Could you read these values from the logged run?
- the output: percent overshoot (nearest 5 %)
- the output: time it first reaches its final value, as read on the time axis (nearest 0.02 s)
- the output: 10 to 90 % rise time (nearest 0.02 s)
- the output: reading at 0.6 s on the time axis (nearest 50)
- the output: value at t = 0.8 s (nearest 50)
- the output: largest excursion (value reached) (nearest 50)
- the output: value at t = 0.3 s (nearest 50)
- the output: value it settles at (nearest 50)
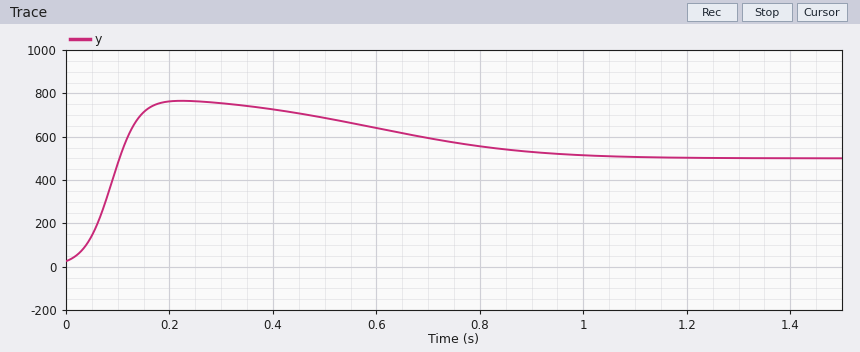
55 %
0.10 s
0.06 s
650
550
750
750
500
